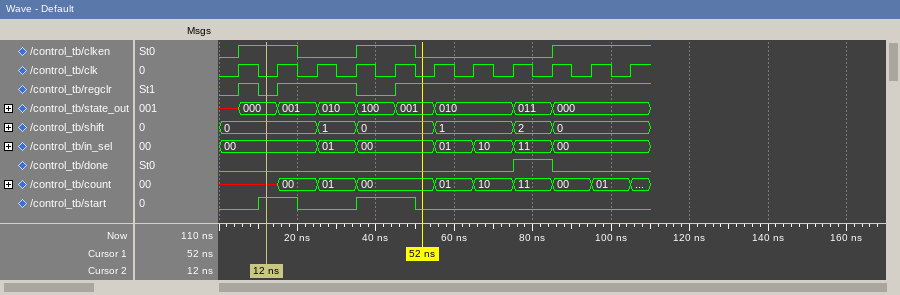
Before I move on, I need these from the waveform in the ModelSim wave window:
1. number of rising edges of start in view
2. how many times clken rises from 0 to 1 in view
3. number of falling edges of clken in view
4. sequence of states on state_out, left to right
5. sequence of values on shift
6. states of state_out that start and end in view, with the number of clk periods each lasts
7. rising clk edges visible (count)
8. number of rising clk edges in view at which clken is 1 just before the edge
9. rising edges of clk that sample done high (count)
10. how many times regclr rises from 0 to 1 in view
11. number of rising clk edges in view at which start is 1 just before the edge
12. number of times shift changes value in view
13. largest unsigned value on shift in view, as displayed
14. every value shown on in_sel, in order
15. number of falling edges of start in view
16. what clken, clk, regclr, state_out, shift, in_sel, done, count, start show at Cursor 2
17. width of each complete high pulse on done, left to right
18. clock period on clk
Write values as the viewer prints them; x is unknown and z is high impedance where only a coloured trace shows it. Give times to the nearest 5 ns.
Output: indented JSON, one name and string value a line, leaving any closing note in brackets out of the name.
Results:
{
  "number of rising edges of start in view": "2",
  "how many times clken rises from 0 to 1 in view": "3",
  "number of falling edges of clken in view": "2",
  "sequence of states on state_out, left to right": "x, 000, 001, 010, 100, 001, 010, 011, 000",
  "sequence of values on shift": "0, 1, 0, 1, 2, 0",
  "states of state_out that start and end in view, with the number of clk periods each lasts": "000: 1, 001: 1, 010: 1, 100: 1, 001: 1, 010: 2, 011: 1",
  "rising clk edges visible": "11",
  "number of rising clk edges in view at which clken is 1 just before the edge": "4",
  "rising edges of clk that sample done high": "1",
  "how many times regclr rises from 0 to 1 in view": "3",
  "number of rising clk edges in view at which start is 1 just before the edge": "2",
  "number of times shift changes value in view": "5",
  "largest unsigned value on shift in view, as displayed": "2",
  "every value shown on in_sel, in order": "00, 01, 00, 01, 10, 11, 00",
  "number of falling edges of start in view": "2",
  "what clken, clk, regclr, state_out, shift, in_sel, done, count, start show at Cursor 2": "clken=1, clk=0, regclr=0, state_out=000, shift=0, in_sel=00, done=0, count=x, start=1",
  "width of each complete high pulse on done, left to right": "10 ns",
  "clock period on clk": "10 ns"
}
